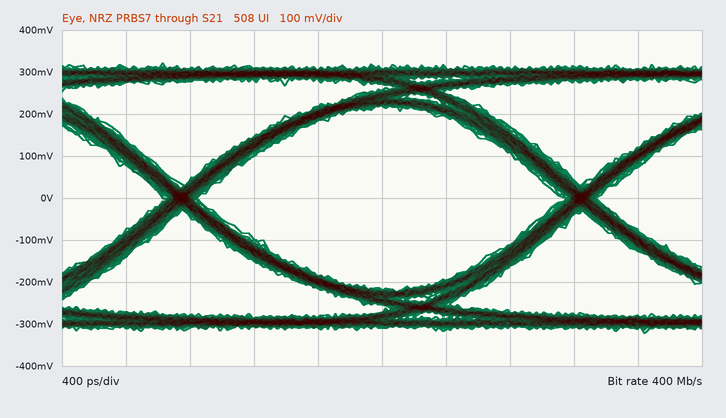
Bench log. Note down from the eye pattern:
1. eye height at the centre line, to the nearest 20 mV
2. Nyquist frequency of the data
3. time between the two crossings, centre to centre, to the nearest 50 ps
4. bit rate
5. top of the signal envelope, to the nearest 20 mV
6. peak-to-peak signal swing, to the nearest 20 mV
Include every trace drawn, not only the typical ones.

440 mV
200 MHz
2.50 ns
400 Mb/s
320 mV
640 mV
